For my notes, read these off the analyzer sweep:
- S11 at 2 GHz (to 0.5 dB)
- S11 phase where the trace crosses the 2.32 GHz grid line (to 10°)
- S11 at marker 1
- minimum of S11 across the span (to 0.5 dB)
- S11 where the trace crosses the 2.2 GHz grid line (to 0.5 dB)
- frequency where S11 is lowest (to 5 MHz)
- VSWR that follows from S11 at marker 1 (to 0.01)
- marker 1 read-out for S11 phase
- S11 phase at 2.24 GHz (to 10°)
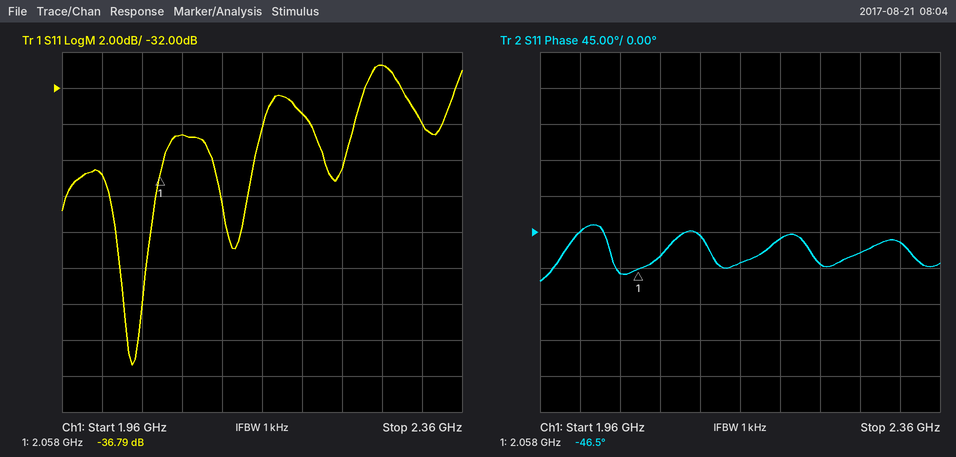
-37.0 dB
-10°
-36.79 dB
-47.5 dB
-33.5 dB
2.030 GHz
1.03
-46.5°
-40°
